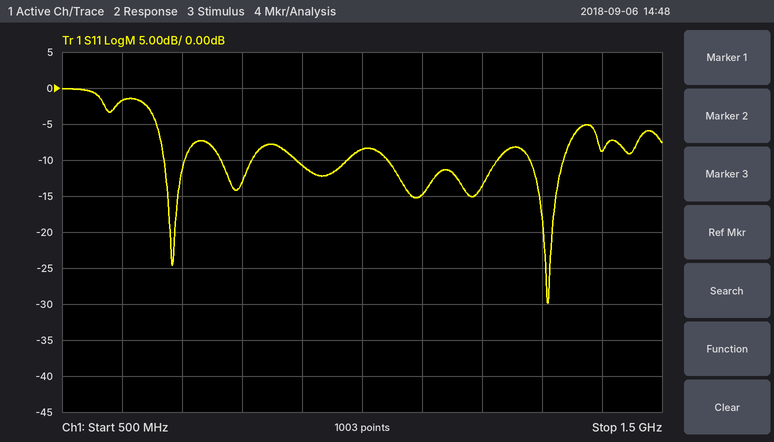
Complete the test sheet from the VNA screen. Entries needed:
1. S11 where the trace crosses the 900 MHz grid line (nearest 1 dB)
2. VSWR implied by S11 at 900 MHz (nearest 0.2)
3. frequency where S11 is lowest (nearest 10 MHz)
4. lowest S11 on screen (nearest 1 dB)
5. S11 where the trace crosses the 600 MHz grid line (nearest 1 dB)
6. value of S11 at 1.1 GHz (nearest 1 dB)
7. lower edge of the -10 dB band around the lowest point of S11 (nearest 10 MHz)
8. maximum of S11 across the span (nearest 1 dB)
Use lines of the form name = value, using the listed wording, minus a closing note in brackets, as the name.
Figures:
S11 where the trace crosses the 900 MHz grid line = -11 dB
VSWR implied by S11 at 900 MHz = 1.8
frequency where S11 is lowest = 1.31 GHz
lowest S11 on screen = -30 dB
S11 where the trace crosses the 600 MHz grid line = -2 dB
value of S11 at 1.1 GHz = -15 dB
lower edge of the -10 dB band around the lowest point of S11 = 1.28 GHz
maximum of S11 across the span = 0 dB
